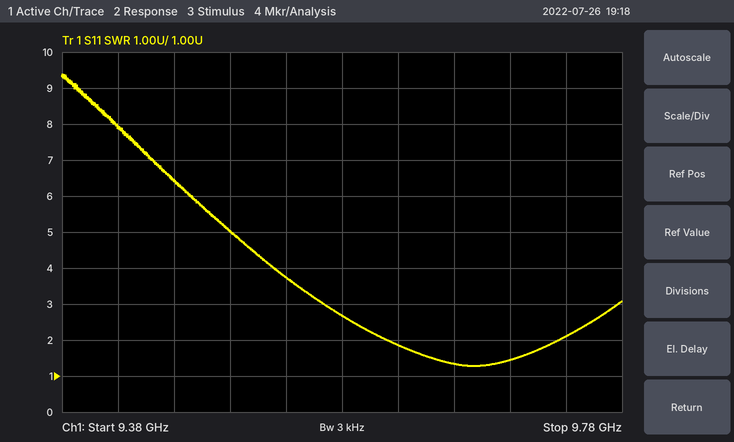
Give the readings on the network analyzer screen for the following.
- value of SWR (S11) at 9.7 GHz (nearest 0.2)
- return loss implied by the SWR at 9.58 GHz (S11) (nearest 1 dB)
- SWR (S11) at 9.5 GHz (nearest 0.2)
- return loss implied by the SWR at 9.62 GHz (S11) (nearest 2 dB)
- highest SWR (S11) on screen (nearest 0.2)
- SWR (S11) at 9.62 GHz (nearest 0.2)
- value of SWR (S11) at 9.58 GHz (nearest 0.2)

1.4
7 dB
5.0
10 dB
9.4
1.8
2.6
